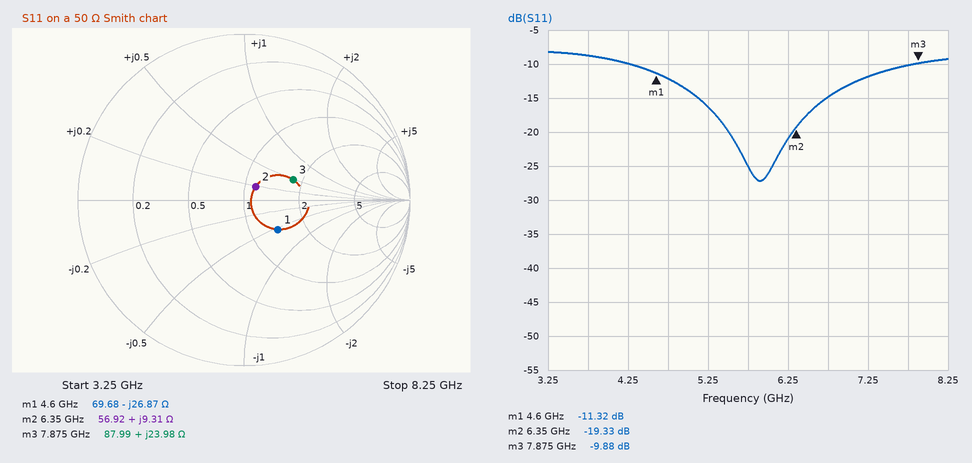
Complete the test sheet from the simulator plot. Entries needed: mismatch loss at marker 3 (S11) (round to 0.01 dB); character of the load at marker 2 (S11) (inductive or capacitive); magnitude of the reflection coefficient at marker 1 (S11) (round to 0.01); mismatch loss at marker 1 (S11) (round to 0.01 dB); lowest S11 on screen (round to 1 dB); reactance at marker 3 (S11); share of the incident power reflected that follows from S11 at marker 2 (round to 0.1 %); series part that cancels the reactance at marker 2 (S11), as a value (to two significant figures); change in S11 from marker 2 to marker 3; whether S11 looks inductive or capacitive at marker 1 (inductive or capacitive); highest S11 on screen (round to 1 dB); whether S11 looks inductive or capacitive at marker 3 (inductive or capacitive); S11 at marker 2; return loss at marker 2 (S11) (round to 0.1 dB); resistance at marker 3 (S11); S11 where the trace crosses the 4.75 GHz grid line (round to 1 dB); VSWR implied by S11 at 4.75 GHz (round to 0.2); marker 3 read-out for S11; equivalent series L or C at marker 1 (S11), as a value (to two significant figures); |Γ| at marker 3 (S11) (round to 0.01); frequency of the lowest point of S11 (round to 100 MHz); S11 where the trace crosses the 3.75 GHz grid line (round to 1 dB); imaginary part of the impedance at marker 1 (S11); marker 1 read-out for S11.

0.47 dB
inductive
0.27
0.33 dB
-27 dB
+23.98 Ω
1.2 %
2.7 pF
9.45 dB
capacitive
-8 dB
inductive
-19.33 dB
19.3 dB
87.99 Ω
-12 dB
1.6
-9.88 dB
1.3 pF
0.32
5.9 GHz
-9 dB
-26.87 Ω
-11.32 dB
